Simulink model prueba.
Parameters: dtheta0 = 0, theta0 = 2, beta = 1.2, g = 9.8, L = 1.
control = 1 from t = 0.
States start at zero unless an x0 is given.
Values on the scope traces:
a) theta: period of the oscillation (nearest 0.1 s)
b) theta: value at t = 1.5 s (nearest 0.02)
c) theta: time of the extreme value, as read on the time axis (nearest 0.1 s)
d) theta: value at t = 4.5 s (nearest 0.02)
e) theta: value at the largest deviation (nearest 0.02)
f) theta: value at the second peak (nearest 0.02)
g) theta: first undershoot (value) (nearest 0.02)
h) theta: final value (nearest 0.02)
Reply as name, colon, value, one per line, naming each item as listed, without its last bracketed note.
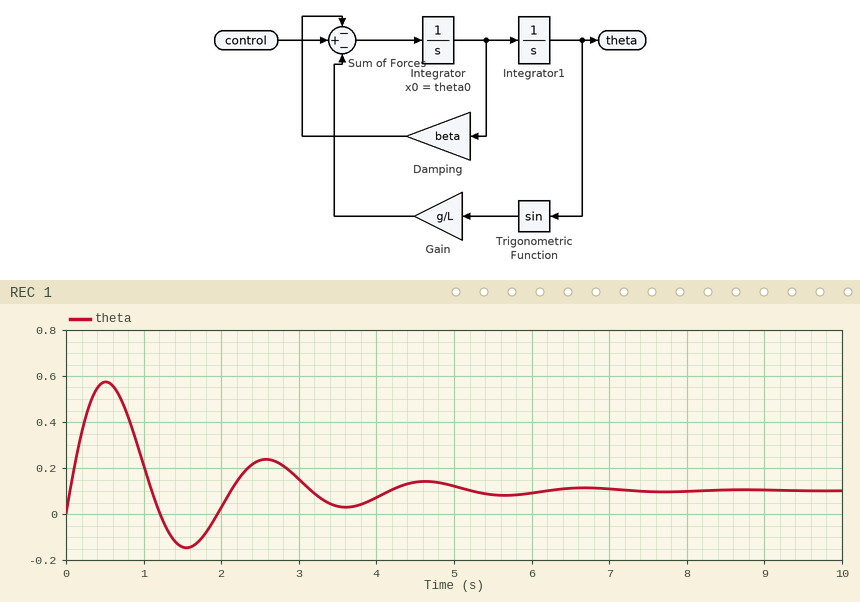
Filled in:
theta: period of the oscillation: 2.1 s
theta: value at t = 1.5 s: -0.14
theta: time of the extreme value, as read on the time axis: 0.5 s
theta: value at t = 4.5 s: 0.14
theta: value at the largest deviation: 0.58
theta: value at the second peak: 0.24
theta: first undershoot (value): -0.14
theta: final value: 0.10
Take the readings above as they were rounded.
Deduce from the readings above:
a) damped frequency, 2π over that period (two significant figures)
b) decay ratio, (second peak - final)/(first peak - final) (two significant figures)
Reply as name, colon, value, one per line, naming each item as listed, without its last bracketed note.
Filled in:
damped frequency, 2π over that period: 3.0 rad/s
decay ratio, (second peak - final)/(first peak - final): 0.29
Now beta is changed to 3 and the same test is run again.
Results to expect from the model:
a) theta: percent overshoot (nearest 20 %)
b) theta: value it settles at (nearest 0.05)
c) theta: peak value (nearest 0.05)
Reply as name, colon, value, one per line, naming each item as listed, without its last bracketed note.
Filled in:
theta: percent overshoot: 300 %
theta: value it settles at: 0.10
theta: peak value: 0.40
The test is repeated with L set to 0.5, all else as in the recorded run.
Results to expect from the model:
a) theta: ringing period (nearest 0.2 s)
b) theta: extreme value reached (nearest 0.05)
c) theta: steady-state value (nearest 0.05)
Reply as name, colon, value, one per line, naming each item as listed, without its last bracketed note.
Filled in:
theta: ringing period: 1.4 s
theta: extreme value reached: 0.40
theta: steady-state value: 0.05
